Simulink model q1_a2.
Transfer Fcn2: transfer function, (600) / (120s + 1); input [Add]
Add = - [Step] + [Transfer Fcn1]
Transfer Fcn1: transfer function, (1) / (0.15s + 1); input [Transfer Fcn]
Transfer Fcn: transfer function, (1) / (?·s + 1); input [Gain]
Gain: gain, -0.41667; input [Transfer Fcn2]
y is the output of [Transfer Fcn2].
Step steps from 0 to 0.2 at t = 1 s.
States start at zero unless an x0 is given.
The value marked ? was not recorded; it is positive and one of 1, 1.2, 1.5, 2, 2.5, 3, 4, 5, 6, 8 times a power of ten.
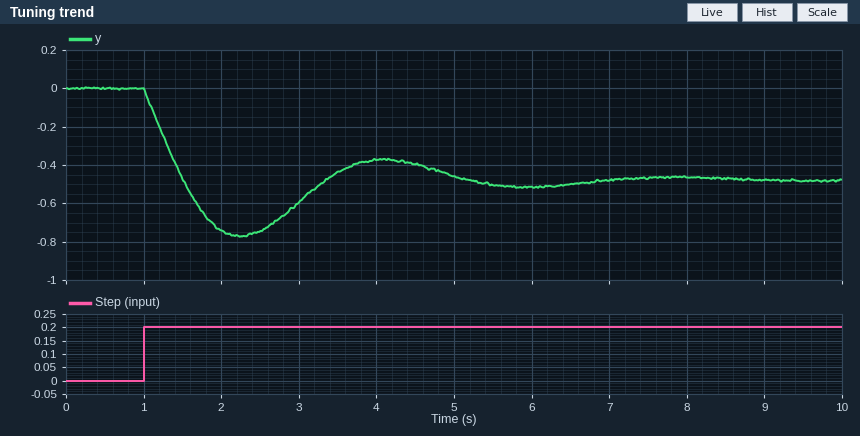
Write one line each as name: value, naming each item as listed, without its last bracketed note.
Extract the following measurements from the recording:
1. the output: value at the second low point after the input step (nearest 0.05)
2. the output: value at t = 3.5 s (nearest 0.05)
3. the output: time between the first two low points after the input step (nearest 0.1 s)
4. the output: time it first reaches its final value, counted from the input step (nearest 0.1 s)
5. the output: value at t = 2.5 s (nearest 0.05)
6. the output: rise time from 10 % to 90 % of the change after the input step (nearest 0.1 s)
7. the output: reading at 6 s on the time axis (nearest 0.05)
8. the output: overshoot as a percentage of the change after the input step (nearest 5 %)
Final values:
the output: value at the second low point after the input step: -0.50
the output: value at t = 3.5 s: -0.45
the output: time between the first two low points after the input step: 3.7 s
the output: time it first reaches its final value, counted from the input step: 0.5 s
the output: value at t = 2.5 s: -0.75
the output: rise time from 10 % to 90 % of the change after the input step: 0.4 s
the output: reading at 6 s on the time axis: -0.50
the output: overshoot as a percentage of the change after the input step: 60 %
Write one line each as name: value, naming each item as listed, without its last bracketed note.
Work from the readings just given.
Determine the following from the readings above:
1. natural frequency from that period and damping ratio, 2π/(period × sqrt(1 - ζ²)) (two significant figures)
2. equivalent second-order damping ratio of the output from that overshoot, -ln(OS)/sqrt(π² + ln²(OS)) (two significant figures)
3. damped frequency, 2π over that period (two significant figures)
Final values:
natural frequency from that period and damping ratio, 2π/(period × sqrt(1 - ζ²)): 1.7 rad/s
equivalent second-order damping ratio of the output from that overshoot, -ln(OS)/sqrt(π² + ln²(OS)): 0.16
damped frequency, 2π over that period: 1.7 rad/s
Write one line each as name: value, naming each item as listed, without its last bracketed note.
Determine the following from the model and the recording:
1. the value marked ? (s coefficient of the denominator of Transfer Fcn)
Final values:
the value marked ?: 0.6
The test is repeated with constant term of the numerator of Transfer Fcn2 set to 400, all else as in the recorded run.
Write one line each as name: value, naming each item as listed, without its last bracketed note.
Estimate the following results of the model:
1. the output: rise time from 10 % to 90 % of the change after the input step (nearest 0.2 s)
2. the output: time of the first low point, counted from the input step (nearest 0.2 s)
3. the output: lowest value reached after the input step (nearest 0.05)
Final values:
the output: rise time from 10 % to 90 % of the change after the input step: 0.6 s
the output: time of the first low point, counted from the input step: 1.6 s
the output: lowest value reached after the input step: -0.65
